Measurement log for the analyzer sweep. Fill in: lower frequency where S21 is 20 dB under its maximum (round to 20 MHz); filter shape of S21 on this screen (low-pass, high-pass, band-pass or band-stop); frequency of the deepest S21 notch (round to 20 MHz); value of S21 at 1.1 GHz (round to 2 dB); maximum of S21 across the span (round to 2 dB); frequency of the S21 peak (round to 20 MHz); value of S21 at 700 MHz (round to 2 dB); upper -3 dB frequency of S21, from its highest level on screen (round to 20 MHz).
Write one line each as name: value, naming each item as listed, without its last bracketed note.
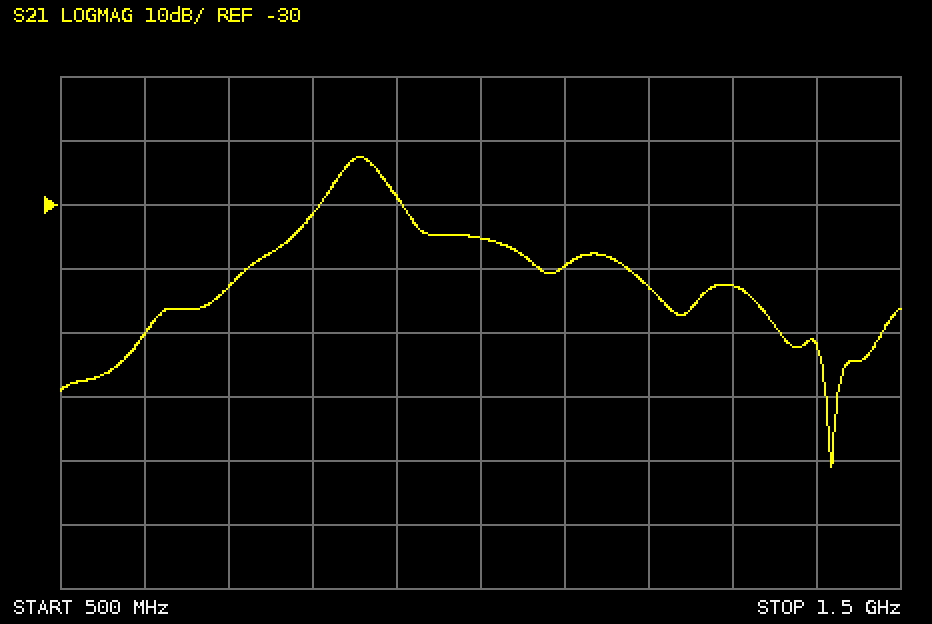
lower frequency where S21 is 20 dB under its maximum: 700 MHz
filter shape of S21 on this screen: band-pass
frequency of the deepest S21 notch: 1.42 GHz
value of S21 at 1.1 GHz: -40 dB
maximum of S21 across the span: -22 dB
frequency of the S21 peak: 860 MHz
value of S21 at 700 MHz: -42 dB
upper -3 dB frequency of S21, from its highest level on screen: 880 MHz
